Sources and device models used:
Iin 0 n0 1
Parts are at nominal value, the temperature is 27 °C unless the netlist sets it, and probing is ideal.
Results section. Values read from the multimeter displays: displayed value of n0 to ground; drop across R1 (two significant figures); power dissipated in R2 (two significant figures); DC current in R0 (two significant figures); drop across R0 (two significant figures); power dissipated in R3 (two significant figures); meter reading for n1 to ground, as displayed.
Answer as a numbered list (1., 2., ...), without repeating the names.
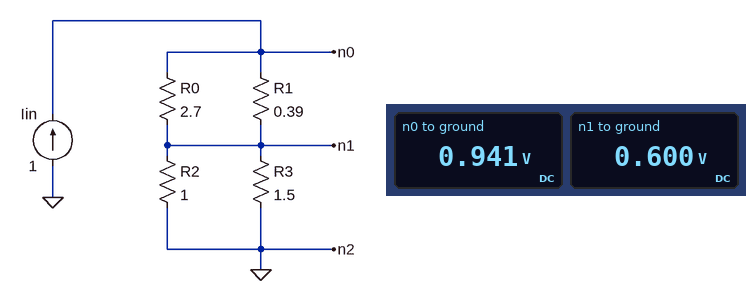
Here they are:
1. 0.941 V
2. 340 mV
3. 360 mW
4. 130 mA
5. 340 mV
6. 240 mW
7. 0.600 V
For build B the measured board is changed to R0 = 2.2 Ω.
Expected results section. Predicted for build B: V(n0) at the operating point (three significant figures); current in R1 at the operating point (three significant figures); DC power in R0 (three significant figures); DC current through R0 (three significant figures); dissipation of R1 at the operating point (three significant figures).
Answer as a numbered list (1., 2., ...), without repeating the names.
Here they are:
1. 931 mV
2. 849 mA
3. 49.9 mW
4. 151 mA
5. 281 mW
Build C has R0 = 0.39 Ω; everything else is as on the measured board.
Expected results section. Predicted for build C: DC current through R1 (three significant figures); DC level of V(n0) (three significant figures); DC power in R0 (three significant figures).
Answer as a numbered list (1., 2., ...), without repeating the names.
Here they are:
1. 500 mA
2. 795 mV
3. 97.5 mW
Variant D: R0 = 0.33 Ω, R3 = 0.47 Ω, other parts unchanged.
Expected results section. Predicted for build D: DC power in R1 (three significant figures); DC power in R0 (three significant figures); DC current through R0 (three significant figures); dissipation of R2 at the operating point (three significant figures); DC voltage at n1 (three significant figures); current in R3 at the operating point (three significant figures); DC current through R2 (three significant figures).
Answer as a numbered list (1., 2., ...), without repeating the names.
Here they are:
1. 81.9 mW
2. 96.8 mW
3. 542 mA
4. 102 mW
5. 320 mV
6. 680 mA
7. 320 mA
